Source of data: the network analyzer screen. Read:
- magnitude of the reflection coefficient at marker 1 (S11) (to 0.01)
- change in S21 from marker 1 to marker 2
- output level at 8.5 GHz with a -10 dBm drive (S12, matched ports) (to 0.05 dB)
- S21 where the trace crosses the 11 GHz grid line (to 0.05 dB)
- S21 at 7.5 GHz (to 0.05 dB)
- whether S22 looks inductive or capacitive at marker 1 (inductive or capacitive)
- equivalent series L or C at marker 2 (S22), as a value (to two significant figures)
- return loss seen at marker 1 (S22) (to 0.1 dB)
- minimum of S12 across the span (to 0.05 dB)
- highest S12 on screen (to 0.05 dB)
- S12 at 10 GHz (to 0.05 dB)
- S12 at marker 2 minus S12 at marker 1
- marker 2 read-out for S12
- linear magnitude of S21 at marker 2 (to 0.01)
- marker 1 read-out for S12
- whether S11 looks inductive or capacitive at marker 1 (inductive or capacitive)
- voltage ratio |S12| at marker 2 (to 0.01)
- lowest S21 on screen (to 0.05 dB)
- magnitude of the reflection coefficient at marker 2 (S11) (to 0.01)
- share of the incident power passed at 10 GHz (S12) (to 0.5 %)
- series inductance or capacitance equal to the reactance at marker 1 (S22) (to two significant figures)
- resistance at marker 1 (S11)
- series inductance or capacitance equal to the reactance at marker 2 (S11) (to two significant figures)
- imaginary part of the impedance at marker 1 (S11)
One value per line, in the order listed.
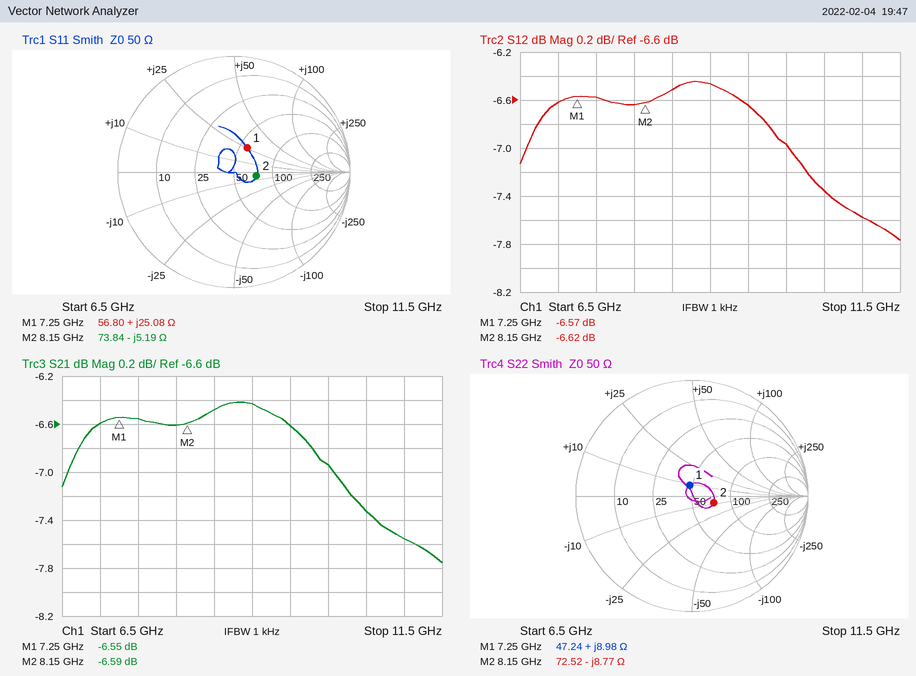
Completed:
0.24
-0.04 dB
-16.50 dBm
-7.55 dB
-6.55 dB
inductive
2.2 pF
20.3 dB
-7.75 dB
-6.45 dB
-6.95 dB
-0.05 dB
-6.62 dB
0.47
-6.57 dB
inductive
0.47
-7.75 dB
0.20
20.0 %
200 pH
56.80 Ω
3.8 pF
+25.08 Ω
